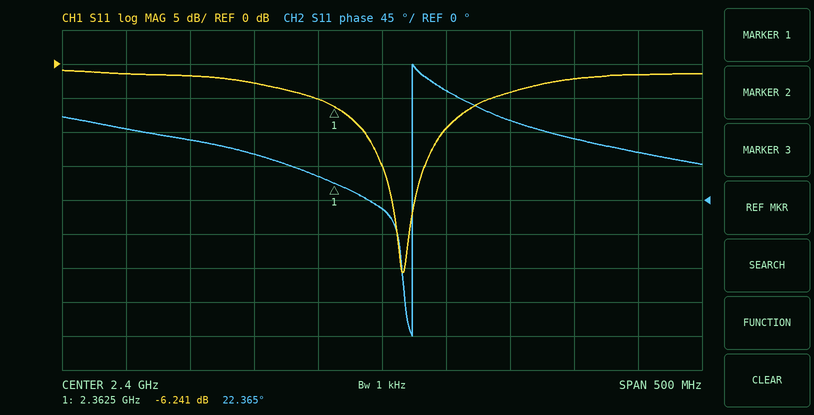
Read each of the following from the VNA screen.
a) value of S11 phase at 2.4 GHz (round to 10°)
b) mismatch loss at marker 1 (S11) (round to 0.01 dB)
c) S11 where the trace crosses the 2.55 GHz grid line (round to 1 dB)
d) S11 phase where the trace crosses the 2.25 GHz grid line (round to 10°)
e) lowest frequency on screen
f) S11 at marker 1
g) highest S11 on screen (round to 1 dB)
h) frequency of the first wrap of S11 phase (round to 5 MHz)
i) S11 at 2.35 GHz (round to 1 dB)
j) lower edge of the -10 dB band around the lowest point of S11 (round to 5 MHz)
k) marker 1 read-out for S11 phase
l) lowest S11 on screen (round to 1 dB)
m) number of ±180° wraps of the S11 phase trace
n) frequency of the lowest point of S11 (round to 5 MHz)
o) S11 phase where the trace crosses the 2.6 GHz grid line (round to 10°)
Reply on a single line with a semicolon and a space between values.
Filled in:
-10°; 1.18 dB; -2 dB; 80°; 2.15 GHz; -6.241 dB; -1 dB; 2.425 GHz; -5 dB; 2.385 GHz; 22.365°; -31 dB; 1; 2.415 GHz; 60°
